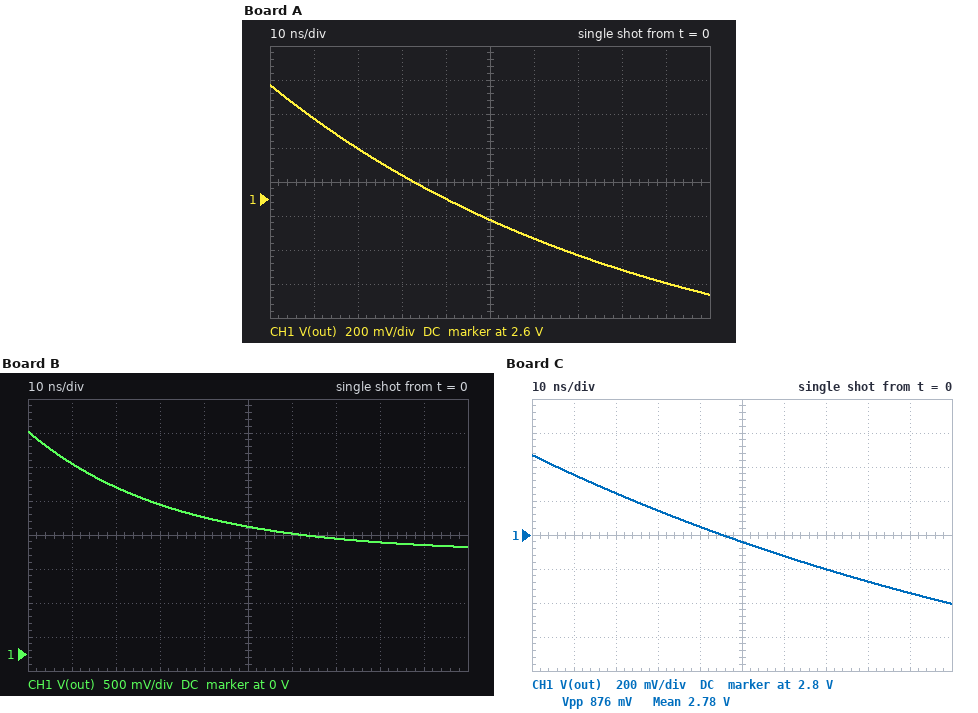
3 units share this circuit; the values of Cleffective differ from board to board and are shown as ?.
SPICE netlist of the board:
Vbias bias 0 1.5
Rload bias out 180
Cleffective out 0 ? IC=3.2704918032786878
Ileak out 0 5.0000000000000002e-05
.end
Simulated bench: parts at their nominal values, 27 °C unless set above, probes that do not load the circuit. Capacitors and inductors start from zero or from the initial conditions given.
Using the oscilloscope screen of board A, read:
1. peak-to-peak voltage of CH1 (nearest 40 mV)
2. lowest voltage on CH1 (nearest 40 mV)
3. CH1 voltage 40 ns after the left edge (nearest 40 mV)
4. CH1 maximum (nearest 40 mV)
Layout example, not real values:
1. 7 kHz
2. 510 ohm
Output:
1. 1.24 V
2. 2.04 V
3. 2.60 V
4. 3.28 V
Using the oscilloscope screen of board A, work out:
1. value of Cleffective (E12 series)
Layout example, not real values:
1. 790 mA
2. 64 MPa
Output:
1. 470 pF
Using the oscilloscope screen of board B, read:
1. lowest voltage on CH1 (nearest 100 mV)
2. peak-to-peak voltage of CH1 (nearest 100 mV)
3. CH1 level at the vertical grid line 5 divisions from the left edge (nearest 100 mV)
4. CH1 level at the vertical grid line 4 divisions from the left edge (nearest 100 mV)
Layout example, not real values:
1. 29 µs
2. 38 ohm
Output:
1. 1.6 V
2. 1.7 V
3. 1.9 V
4. 2.0 V
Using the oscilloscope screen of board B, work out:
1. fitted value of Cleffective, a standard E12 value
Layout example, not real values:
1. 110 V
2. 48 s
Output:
1. 180 pF
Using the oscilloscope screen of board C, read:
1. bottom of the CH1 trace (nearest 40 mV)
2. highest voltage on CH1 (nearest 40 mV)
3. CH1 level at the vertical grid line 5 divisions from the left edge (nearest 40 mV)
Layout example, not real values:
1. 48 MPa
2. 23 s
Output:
1. 2.40 V
2. 3.28 V
3. 2.76 V
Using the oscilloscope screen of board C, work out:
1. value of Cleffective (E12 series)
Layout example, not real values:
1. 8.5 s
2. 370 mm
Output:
1. 820 pF
